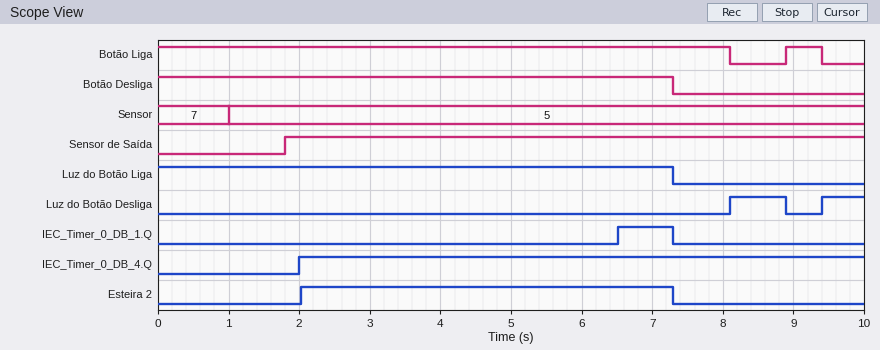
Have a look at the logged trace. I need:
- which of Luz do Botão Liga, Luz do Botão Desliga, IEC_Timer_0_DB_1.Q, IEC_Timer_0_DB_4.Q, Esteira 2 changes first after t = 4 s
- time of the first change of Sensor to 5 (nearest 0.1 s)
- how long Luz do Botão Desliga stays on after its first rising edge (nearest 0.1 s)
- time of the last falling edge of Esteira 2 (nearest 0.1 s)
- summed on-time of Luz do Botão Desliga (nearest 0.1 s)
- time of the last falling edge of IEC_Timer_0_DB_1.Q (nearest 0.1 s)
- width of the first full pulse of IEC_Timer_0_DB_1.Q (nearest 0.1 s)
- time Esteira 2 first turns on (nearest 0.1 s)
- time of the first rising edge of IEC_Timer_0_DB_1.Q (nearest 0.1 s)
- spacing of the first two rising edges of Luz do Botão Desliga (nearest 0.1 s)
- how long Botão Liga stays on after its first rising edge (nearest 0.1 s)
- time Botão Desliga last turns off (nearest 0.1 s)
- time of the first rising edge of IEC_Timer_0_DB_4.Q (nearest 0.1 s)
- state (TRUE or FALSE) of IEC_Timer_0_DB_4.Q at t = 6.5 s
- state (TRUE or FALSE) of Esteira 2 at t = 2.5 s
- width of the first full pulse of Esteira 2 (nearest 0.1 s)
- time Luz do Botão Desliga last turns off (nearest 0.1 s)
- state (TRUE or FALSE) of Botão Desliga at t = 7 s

IEC_Timer_0_DB_1.Q
1.0 s
0.8 s
7.3 s
1.4 s
7.3 s
0.8 s
2.0 s
6.5 s
1.3 s
0.5 s
7.3 s
2.0 s
TRUE
TRUE
5.3 s
8.9 s
TRUE
